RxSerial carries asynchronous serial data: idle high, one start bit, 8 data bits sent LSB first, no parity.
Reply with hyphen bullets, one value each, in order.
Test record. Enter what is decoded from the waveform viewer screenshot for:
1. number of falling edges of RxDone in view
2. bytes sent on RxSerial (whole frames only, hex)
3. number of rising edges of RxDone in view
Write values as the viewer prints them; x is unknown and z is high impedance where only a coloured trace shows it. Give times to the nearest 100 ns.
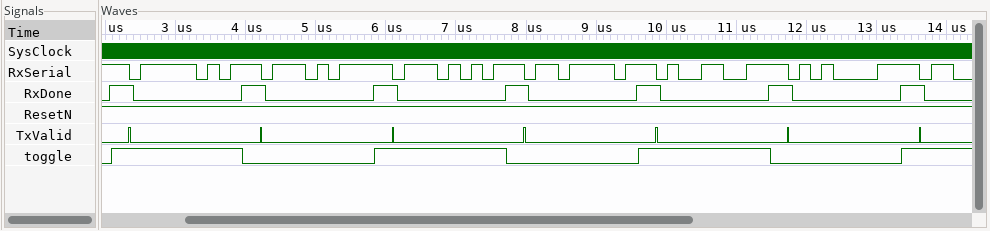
- 7
- 5F, D7, 57, 7B, 99, 85
- 7
